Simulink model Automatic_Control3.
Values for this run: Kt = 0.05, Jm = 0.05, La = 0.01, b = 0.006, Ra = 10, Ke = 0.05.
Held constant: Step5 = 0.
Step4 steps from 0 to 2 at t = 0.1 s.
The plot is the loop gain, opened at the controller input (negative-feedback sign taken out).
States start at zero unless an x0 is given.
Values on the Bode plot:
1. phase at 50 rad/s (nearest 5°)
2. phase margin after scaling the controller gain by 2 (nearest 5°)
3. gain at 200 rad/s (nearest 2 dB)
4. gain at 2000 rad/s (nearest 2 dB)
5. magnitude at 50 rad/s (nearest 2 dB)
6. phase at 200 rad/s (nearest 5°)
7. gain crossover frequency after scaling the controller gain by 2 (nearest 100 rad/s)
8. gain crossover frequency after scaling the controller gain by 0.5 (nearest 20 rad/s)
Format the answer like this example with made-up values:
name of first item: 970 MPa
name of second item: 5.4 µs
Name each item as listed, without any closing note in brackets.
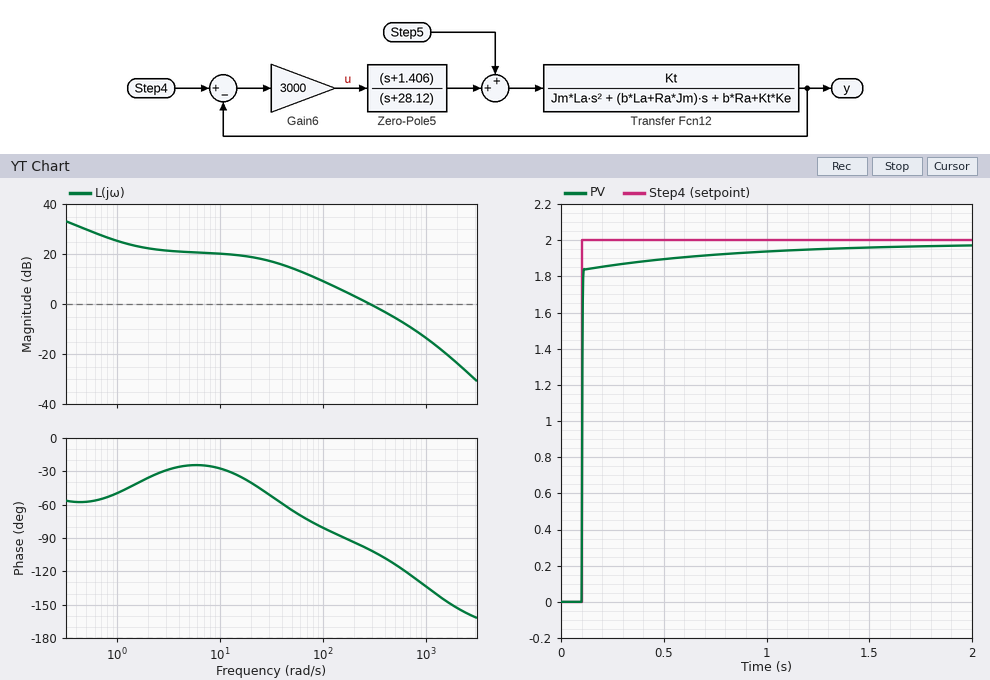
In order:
phase at 50 rad/s: -65°
phase margin after scaling the controller gain by 2: 65°
gain at 200 rad/s: 4 dB
gain at 2000 rad/s: -24 dB
magnitude at 50 rad/s: 14 dB
phase at 200 rad/s: -95°
gain crossover frequency after scaling the controller gain by 2: 500 rad/s
gain crossover frequency after scaling the controller gain by 0.5: 140 rad/s
